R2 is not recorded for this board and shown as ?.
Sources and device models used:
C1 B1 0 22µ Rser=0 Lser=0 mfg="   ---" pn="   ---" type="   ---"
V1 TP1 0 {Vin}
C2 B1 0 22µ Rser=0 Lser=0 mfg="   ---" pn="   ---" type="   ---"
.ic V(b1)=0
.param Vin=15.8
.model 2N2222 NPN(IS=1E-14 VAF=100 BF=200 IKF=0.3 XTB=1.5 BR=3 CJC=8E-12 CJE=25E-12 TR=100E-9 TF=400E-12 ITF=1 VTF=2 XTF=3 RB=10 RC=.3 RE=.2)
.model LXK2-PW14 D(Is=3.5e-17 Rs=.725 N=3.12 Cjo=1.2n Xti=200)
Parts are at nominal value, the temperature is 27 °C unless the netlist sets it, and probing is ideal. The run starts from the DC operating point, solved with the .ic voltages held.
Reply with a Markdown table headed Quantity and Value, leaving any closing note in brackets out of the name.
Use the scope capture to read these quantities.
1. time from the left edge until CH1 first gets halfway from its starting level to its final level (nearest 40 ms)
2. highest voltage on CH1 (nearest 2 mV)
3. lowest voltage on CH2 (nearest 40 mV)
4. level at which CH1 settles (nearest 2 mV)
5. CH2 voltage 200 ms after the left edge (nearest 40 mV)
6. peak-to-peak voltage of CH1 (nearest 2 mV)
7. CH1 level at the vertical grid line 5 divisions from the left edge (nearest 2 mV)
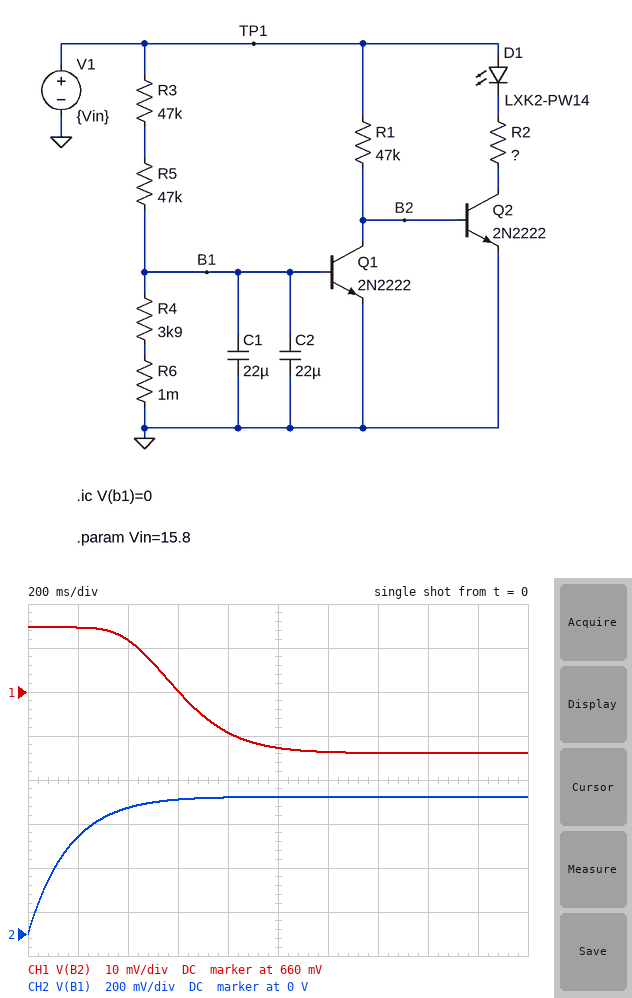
| Quantity | Value |
|---|---|
| time from the left edge until CH1 first gets halfway from its starting level to its final level | 600 ms |
| highest voltage on CH1 | 674 mV |
| lowest voltage on CH2 | 0 V |
| level at which CH1 settles | 646 mV |
| CH2 voltage 200 ms after the left edge | 440 mV |
| peak-to-peak voltage of CH1 | 28 mV |
| CH1 level at the vertical grid line 5 divisions from the left edge | 648 mV |
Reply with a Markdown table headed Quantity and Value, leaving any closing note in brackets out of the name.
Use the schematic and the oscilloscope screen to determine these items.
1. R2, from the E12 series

| Quantity | Value |
|---|---|
| R2, from the E12 series | 22 kΩ |
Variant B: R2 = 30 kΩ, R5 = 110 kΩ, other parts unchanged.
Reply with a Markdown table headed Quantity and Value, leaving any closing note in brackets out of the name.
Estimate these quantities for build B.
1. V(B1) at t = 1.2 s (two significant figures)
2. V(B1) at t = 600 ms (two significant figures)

| Quantity | Value |
|---|---|
| V(B1) at t = 1.2 s | 380 mV |
| V(B1) at t = 600 ms | 370 mV |
